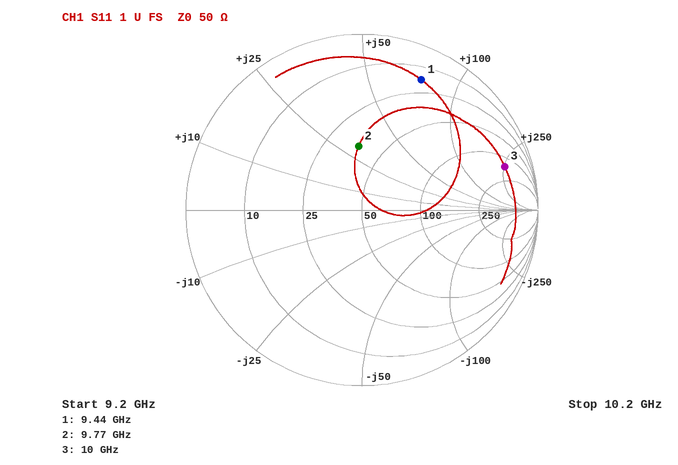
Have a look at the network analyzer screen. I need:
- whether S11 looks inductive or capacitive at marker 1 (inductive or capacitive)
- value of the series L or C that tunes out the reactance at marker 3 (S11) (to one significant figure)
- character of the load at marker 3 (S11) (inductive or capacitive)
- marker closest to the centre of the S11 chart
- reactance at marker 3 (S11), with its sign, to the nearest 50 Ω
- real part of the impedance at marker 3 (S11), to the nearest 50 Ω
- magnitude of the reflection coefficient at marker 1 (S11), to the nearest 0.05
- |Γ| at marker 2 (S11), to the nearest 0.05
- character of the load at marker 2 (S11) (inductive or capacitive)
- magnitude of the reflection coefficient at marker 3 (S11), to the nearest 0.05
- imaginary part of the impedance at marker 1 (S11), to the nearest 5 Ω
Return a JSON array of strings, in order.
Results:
["inductive", "60 fF", "inductive", "marker 2", "+250 Ω", "150 Ω", "0.80", "0.35", "inductive", "0.85", "+75 Ω"]
